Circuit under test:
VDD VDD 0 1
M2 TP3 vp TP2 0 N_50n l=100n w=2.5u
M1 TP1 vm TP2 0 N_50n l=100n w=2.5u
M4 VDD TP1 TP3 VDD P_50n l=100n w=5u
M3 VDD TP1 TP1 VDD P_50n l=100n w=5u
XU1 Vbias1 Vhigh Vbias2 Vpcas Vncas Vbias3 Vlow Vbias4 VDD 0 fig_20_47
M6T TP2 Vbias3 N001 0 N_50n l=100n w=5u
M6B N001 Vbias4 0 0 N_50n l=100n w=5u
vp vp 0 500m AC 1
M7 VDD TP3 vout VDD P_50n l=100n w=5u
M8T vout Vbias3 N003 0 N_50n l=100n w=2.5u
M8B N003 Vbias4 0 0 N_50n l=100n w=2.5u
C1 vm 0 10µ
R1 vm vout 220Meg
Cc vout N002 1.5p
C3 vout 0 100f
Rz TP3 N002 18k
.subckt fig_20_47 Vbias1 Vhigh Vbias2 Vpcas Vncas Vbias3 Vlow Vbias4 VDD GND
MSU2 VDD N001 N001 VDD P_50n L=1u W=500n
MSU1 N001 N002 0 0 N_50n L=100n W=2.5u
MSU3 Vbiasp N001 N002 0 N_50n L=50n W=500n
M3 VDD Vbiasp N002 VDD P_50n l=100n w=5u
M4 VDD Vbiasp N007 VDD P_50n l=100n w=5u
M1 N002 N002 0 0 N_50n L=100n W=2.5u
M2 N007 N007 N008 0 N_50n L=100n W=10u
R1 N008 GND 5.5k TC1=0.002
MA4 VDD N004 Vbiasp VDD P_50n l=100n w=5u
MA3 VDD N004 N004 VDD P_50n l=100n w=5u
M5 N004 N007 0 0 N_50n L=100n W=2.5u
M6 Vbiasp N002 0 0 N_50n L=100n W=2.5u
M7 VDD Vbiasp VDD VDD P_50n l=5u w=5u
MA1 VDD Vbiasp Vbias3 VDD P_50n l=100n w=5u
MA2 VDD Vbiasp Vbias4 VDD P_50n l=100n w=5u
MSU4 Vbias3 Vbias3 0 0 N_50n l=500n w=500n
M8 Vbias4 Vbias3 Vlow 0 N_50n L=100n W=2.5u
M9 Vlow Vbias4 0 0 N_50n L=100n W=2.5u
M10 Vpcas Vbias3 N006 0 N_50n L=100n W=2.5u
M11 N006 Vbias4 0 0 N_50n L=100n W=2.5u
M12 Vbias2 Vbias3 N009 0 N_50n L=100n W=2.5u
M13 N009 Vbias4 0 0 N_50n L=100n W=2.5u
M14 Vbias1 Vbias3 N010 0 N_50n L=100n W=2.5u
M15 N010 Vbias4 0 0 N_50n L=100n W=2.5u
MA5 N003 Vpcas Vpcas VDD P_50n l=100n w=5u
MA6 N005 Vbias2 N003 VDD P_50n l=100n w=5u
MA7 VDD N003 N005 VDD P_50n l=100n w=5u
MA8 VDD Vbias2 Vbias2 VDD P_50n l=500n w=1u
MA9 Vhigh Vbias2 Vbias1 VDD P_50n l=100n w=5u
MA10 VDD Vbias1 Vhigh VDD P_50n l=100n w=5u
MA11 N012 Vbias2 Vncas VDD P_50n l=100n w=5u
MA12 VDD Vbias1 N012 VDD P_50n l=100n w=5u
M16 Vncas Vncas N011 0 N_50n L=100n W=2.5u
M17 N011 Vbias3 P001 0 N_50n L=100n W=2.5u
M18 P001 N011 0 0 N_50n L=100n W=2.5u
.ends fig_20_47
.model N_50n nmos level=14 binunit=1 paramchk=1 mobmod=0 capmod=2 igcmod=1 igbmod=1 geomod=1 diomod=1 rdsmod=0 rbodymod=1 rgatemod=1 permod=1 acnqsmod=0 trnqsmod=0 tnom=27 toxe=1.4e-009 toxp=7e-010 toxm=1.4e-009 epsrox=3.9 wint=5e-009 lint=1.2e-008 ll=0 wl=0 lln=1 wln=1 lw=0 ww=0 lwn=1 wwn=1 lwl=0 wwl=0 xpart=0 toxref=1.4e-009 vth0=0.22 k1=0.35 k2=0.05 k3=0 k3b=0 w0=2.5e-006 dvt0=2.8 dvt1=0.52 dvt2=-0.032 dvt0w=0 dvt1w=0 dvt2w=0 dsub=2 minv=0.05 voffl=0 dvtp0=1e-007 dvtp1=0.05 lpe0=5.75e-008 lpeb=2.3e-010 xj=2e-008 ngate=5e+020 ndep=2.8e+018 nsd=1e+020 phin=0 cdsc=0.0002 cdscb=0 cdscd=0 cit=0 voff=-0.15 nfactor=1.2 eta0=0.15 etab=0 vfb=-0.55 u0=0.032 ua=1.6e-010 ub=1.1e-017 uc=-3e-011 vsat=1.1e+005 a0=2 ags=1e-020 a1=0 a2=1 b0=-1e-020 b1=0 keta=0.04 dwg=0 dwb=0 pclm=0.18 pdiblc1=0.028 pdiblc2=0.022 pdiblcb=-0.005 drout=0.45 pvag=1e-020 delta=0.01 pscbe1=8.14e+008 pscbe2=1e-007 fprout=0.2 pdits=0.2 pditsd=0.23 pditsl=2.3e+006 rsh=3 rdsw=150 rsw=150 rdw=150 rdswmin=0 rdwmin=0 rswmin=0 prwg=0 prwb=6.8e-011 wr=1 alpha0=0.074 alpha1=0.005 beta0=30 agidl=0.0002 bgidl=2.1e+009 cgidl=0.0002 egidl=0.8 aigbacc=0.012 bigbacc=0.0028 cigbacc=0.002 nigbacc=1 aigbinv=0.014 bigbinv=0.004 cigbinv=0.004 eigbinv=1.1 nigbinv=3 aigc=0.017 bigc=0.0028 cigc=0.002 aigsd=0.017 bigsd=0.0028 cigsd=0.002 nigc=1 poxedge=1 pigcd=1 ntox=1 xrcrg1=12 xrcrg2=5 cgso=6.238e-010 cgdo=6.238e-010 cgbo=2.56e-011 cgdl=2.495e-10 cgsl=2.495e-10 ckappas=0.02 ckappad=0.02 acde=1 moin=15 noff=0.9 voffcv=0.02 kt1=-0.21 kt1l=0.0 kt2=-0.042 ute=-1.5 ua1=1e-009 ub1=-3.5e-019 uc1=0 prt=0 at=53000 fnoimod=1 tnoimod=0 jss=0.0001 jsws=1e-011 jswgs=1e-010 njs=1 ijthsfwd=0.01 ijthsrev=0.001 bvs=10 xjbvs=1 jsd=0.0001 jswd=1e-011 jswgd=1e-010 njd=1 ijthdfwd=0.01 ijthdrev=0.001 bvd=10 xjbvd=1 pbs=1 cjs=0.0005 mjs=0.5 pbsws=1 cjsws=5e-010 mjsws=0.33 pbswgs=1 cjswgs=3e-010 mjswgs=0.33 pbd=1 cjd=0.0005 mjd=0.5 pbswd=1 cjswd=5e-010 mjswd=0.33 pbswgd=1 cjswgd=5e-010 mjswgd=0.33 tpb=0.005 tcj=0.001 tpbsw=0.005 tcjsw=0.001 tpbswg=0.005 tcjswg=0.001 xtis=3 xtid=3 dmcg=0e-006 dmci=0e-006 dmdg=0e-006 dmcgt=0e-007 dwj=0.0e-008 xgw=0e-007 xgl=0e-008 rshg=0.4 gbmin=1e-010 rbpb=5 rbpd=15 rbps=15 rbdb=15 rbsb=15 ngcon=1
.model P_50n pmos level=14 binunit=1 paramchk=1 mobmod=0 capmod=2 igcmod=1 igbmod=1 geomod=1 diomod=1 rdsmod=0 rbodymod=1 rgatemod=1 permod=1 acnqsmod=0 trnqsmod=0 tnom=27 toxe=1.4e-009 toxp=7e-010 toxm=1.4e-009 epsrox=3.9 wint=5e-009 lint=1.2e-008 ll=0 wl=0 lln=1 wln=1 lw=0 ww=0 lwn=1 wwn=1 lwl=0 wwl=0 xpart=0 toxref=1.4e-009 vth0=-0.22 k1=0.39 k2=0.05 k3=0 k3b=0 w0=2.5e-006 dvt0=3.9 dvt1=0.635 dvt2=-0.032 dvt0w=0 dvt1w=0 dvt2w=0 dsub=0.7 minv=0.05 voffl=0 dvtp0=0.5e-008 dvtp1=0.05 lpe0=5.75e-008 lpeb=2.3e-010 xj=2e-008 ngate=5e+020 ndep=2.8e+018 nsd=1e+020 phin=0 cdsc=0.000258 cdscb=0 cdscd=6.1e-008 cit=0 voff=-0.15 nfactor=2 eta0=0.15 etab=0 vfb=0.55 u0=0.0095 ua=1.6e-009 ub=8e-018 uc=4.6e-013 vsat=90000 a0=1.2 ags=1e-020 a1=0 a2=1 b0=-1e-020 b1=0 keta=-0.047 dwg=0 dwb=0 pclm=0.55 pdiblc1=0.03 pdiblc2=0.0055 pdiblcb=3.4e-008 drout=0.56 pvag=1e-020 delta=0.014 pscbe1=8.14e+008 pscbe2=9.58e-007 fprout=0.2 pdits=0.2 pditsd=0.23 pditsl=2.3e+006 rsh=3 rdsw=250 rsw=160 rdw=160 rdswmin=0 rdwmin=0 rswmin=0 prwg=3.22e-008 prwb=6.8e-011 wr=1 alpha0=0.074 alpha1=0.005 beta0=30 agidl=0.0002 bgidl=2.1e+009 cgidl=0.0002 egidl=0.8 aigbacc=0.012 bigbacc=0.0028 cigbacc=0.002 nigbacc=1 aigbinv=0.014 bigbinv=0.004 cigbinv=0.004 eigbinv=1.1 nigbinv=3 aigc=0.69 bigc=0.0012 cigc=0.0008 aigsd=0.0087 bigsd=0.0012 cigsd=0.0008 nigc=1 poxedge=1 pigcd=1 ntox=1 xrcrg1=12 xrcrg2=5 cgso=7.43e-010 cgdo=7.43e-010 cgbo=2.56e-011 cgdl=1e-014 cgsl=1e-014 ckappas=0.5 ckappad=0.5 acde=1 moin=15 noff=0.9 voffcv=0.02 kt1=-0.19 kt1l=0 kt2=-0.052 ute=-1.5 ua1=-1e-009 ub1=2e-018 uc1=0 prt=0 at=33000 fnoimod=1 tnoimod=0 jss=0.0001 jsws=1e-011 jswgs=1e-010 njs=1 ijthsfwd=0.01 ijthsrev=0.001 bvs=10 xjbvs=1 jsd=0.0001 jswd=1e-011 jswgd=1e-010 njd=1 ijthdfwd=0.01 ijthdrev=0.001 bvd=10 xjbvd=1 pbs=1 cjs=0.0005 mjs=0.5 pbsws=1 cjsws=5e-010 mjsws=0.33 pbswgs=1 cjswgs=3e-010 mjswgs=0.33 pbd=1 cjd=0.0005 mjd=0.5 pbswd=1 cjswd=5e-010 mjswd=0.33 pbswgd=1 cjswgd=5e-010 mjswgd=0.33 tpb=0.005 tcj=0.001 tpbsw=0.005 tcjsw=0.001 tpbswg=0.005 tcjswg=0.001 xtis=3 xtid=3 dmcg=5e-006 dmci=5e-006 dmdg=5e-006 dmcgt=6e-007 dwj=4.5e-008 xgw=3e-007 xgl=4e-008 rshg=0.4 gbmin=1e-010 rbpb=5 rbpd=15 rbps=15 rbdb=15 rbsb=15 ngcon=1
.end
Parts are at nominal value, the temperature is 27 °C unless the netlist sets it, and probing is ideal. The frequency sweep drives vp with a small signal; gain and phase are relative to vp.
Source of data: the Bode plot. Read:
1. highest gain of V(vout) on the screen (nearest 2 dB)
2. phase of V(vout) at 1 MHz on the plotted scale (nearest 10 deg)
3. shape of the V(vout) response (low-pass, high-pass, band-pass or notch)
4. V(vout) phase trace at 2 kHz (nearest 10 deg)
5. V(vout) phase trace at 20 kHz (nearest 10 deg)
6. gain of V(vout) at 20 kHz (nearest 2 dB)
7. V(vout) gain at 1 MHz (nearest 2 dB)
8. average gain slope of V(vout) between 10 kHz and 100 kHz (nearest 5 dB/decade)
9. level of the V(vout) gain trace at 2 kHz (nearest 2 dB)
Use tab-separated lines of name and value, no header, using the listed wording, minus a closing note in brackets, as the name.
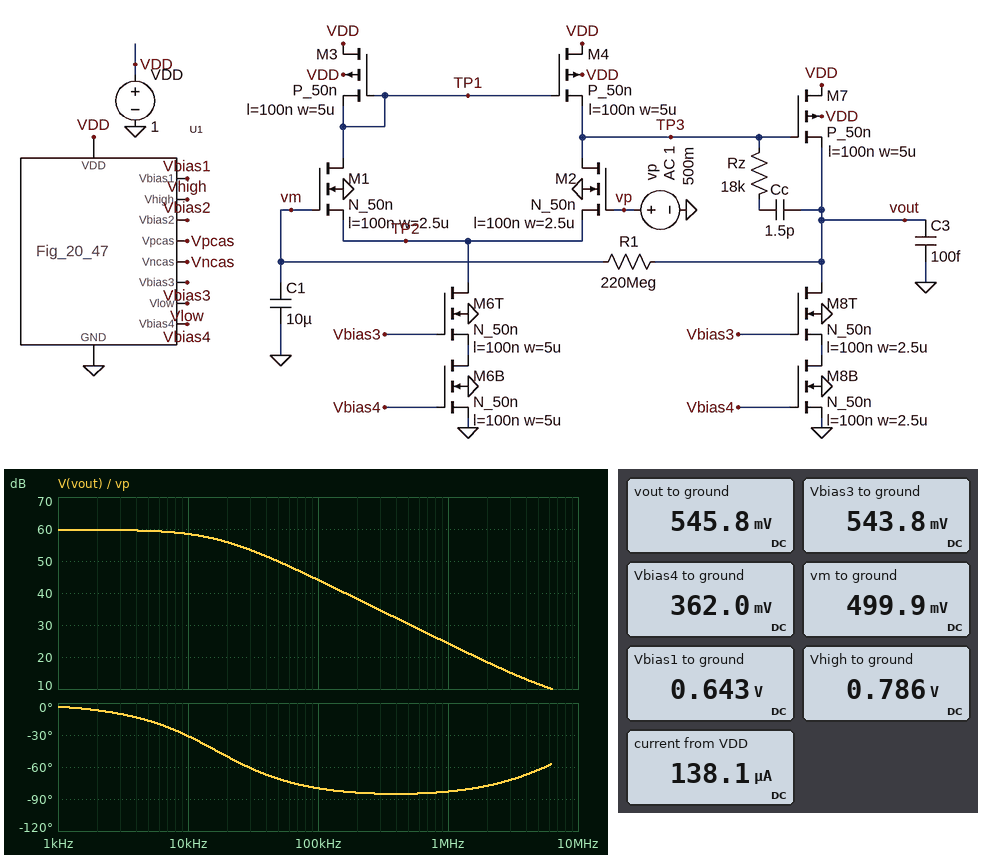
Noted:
highest gain of V(vout) on the screen	60 dB
phase of V(vout) at 1 MHz on the plotted scale	-80 deg
shape of the V(vout) response	low-pass
V(vout) phase trace at 2 kHz	-10 deg
V(vout) phase trace at 20 kHz	-50 deg
gain of V(vout) at 20 kHz	56 dB
V(vout) gain at 1 MHz	24 dB
average gain slope of V(vout) between 10 kHz and 100 kHz	-15 dB/decade
level of the V(vout) gain trace at 2 kHz	60 dB
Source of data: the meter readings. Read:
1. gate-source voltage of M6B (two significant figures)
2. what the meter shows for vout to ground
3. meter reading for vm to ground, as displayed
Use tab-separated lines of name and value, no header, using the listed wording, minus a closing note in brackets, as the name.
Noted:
gate-source voltage of M6B	360 mV
what the meter shows for vout to ground	545.8 mV
meter reading for vm to ground, as displayed	499.9 mV
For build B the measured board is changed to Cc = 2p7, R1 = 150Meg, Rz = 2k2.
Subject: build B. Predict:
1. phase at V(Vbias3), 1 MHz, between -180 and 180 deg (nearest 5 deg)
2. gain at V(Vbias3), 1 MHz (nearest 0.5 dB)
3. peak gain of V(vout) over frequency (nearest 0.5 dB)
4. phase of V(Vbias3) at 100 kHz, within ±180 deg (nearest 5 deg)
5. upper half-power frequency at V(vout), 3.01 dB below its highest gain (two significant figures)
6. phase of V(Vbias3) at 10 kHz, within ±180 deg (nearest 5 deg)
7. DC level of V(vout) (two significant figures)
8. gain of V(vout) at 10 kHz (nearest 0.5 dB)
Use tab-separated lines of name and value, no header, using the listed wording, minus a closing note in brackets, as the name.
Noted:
phase at V(Vbias3), 1 MHz, between -180 and 180 deg	10 deg
gain at V(Vbias3), 1 MHz	-50.5 dB
peak gain of V(vout) over frequency	60.0 dB
phase of V(Vbias3) at 100 kHz, within ±180 deg	5 deg
upper half-power frequency at V(vout), 3.01 dB below its highest gain	9.2 kHz
phase of V(Vbias3) at 10 kHz, within ±180 deg	20 deg
DC level of V(vout)	530 mV
gain of V(vout) at 10 kHz	56.5 dB
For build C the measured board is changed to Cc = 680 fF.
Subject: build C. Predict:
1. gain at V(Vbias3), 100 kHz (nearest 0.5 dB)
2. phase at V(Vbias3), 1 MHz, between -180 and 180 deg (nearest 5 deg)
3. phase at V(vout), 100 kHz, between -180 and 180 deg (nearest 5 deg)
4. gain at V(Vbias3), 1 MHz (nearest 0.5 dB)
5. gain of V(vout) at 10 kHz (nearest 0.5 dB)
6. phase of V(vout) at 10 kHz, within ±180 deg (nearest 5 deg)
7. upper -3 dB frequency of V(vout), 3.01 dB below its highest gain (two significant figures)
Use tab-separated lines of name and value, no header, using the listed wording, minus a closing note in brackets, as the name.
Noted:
gain at V(Vbias3), 100 kHz	-39.5 dB
phase at V(Vbias3), 1 MHz, between -180 and 180 deg	5 deg
phase at V(vout), 100 kHz, between -180 and 180 deg	-70 deg
gain at V(Vbias3), 1 MHz	-39.0 dB
gain of V(vout) at 10 kHz	59.5 dB
phase of V(vout) at 10 kHz, within ±180 deg	-15 deg
upper -3 dB frequency of V(vout), 3.01 dB below its highest gain	36 kHz
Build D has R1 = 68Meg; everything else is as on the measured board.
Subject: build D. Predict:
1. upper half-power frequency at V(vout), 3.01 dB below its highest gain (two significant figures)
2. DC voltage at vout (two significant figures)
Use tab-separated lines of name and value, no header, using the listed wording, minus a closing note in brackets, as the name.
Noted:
upper half-power frequency at V(vout), 3.01 dB below its highest gain	16 kHz
DC voltage at vout	510 mV
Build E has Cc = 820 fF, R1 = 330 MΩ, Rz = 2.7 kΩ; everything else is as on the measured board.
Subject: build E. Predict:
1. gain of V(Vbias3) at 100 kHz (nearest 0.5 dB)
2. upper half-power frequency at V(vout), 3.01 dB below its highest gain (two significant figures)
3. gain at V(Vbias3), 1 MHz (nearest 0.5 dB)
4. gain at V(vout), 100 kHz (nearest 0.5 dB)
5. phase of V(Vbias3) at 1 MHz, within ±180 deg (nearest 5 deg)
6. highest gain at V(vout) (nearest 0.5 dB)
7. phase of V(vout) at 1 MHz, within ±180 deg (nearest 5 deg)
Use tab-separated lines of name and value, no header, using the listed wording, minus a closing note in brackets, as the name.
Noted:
gain of V(Vbias3) at 100 kHz	-41.0 dB
upper half-power frequency at V(vout), 3.01 dB below its highest gain	31 kHz
gain at V(Vbias3), 1 MHz	-40.5 dB
gain at V(vout), 100 kHz	49.0 dB
phase of V(Vbias3) at 1 MHz, within ±180 deg	5 deg
highest gain at V(vout)	59.5 dB
phase of V(vout) at 1 MHz, within ±180 deg	-90 deg
